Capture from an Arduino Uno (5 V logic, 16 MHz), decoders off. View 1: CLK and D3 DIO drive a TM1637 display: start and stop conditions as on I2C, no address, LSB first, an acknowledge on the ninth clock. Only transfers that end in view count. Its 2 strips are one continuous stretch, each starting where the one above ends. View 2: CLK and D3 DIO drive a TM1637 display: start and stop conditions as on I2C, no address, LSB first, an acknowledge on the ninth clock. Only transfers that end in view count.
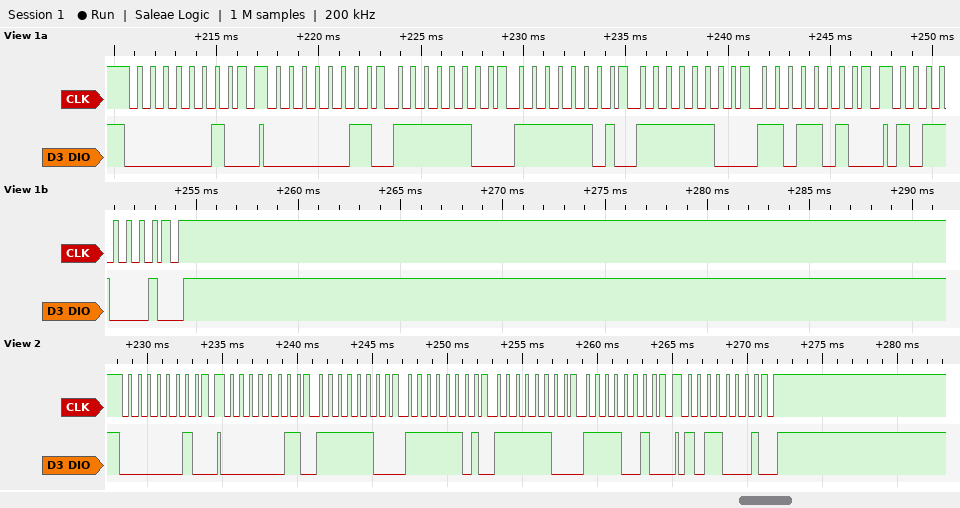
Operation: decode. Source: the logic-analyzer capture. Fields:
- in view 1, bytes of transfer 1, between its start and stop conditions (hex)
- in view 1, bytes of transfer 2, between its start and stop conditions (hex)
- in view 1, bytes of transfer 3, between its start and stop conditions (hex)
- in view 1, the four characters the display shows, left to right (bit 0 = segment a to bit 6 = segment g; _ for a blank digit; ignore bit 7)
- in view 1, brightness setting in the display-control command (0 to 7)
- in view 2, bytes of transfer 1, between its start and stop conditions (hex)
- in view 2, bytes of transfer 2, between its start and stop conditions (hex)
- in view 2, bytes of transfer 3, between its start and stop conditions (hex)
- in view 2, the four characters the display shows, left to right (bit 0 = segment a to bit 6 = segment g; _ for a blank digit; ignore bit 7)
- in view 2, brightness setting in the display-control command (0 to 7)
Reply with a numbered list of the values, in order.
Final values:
1. 40
2. C0 3F BF 3F 5B
3. 8D
4. 0002
5. 5
6. 40
7. C0 3F BF 3F 4F
8. 8D
9. 0003
10. 5
